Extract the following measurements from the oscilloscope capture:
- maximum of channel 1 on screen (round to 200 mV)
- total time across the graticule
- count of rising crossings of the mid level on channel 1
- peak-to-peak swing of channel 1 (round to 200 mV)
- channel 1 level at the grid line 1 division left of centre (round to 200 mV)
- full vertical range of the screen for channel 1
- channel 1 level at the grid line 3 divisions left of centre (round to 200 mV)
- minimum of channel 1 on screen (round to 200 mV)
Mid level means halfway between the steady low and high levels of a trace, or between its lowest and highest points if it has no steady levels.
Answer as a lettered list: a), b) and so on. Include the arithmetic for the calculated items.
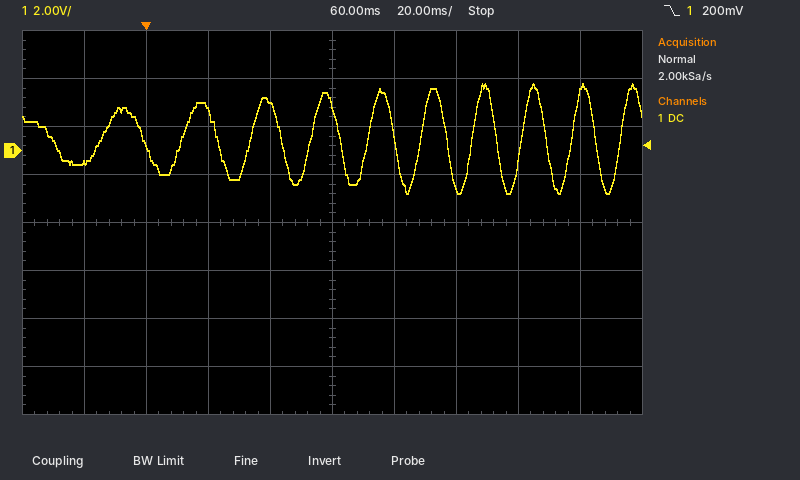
a) 2.8 V
b) 200 ms
c) 10
d) 2.8 V − (-1.8 V) = 4.6 V
e) 2.0 V
f) 16 V
g) 200 mV
h) -1.8 V
